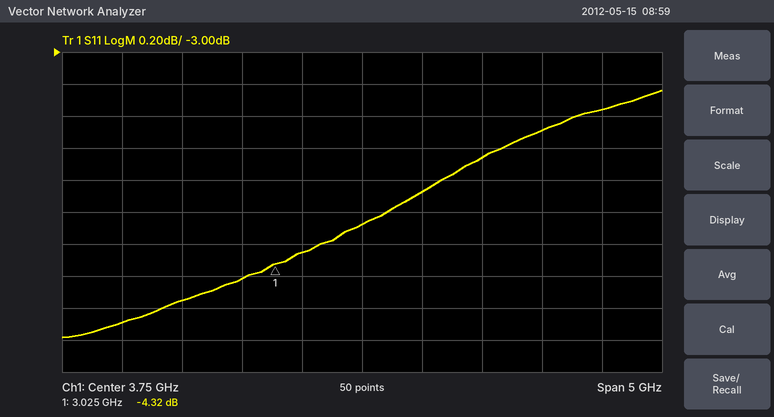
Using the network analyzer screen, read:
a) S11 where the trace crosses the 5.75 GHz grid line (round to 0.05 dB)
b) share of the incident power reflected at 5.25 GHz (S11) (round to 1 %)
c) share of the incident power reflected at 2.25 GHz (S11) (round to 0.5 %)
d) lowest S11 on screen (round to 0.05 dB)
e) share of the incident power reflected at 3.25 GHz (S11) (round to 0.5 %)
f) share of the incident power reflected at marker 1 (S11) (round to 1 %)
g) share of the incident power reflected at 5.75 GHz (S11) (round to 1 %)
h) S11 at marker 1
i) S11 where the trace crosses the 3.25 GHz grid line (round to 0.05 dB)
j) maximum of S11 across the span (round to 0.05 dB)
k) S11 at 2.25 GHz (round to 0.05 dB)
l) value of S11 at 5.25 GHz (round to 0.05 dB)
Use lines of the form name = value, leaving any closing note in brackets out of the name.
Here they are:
S11 where the trace crosses the 5.75 GHz grid line = -3.35 dB
share of the incident power reflected at 5.25 GHz (S11) = 45 %
share of the incident power reflected at 2.25 GHz (S11) = 35.0 %
lowest S11 on screen = -4.80 dB
share of the incident power reflected at 3.25 GHz (S11) = 37.5 %
share of the incident power reflected at marker 1 (S11) = 37 %
share of the incident power reflected at 5.75 GHz (S11) = 46 %
S11 at marker 1 = -4.32 dB
S11 where the trace crosses the 3.25 GHz grid line = -4.25 dB
maximum of S11 across the span = -3.25 dB
S11 at 2.25 GHz = -4.55 dB
value of S11 at 5.25 GHz = -3.50 dB
